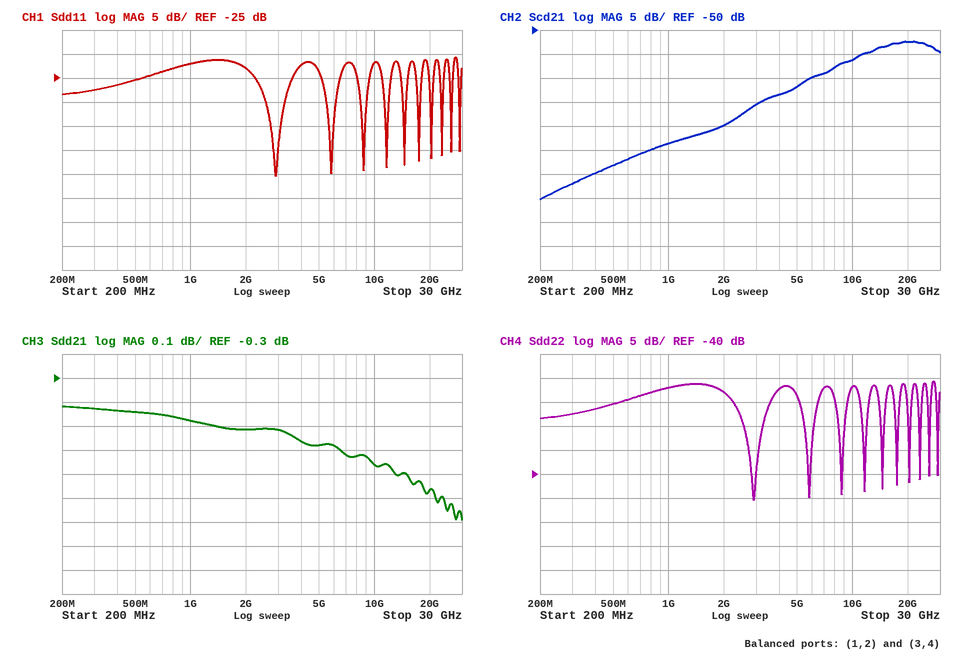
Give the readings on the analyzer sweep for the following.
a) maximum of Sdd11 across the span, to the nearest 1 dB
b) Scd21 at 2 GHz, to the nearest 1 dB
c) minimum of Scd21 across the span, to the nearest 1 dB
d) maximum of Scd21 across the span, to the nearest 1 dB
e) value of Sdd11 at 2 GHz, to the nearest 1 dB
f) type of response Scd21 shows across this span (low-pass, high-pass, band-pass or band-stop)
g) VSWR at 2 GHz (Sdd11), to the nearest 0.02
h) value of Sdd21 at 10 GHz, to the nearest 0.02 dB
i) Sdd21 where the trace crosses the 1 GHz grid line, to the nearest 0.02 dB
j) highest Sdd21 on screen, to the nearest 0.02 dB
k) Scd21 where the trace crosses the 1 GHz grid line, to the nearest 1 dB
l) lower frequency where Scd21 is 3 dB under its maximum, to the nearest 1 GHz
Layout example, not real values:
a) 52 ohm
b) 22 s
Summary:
a) -21 dB
b) -70 dB
c) -85 dB
d) -52 dB
e) -23 dB
f) high-pass
g) 1.16
h) -0.66 dB
i) -0.48 dB
j) -0.42 dB
k) -74 dB
l) 11 GHz
